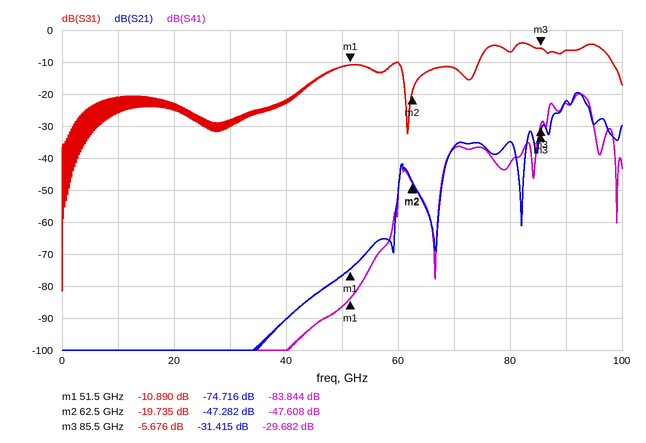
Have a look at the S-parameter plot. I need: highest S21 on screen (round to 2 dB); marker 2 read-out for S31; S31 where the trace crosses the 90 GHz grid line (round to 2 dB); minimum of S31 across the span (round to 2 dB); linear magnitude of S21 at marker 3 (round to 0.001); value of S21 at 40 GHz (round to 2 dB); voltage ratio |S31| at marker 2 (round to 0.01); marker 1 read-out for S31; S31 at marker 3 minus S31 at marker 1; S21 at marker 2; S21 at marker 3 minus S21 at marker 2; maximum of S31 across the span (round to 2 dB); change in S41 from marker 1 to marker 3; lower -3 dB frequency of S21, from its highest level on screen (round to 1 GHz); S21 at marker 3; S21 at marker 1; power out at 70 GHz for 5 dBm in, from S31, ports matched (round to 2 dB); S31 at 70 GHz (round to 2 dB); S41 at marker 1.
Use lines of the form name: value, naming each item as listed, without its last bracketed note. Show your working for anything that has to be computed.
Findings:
highest S21 on screen: -20 dB
marker 2 read-out for S31: -19.735 dB
S31 where the trace crosses the 90 GHz grid line: -6 dB
minimum of S31 across the span: -82 dB
linear magnitude of S21 at marker 3: 10^(-31.415/20) ≈ 0.027
value of S21 at 40 GHz: -90 dB
voltage ratio |S31| at marker 2: 10^(-19.735/20) ≈ 0.10
marker 1 read-out for S31: -10.890 dB
S31 at marker 3 minus S31 at marker 1: -5.676 − (-10.89) = 5.214 dB
S21 at marker 2: -47.282 dB
S21 at marker 3 minus S21 at marker 2: -31.415 − (-47.282) = 15.867 dB
maximum of S31 across the span: -4 dB
change in S41 from marker 1 to marker 3: -29.682 − (-83.844) = 54.162 dB
lower -3 dB frequency of S21, from its highest level on screen: 91 GHz
S21 at marker 3: -31.415 dB
S21 at marker 1: -74.716 dB
power out at 70 GHz for 5 dBm in, from S31, ports matched: 5 dBm + (-12 dB) = -6 dBm
S31 at 70 GHz: -12 dB
S41 at marker 1: -83.844 dB
